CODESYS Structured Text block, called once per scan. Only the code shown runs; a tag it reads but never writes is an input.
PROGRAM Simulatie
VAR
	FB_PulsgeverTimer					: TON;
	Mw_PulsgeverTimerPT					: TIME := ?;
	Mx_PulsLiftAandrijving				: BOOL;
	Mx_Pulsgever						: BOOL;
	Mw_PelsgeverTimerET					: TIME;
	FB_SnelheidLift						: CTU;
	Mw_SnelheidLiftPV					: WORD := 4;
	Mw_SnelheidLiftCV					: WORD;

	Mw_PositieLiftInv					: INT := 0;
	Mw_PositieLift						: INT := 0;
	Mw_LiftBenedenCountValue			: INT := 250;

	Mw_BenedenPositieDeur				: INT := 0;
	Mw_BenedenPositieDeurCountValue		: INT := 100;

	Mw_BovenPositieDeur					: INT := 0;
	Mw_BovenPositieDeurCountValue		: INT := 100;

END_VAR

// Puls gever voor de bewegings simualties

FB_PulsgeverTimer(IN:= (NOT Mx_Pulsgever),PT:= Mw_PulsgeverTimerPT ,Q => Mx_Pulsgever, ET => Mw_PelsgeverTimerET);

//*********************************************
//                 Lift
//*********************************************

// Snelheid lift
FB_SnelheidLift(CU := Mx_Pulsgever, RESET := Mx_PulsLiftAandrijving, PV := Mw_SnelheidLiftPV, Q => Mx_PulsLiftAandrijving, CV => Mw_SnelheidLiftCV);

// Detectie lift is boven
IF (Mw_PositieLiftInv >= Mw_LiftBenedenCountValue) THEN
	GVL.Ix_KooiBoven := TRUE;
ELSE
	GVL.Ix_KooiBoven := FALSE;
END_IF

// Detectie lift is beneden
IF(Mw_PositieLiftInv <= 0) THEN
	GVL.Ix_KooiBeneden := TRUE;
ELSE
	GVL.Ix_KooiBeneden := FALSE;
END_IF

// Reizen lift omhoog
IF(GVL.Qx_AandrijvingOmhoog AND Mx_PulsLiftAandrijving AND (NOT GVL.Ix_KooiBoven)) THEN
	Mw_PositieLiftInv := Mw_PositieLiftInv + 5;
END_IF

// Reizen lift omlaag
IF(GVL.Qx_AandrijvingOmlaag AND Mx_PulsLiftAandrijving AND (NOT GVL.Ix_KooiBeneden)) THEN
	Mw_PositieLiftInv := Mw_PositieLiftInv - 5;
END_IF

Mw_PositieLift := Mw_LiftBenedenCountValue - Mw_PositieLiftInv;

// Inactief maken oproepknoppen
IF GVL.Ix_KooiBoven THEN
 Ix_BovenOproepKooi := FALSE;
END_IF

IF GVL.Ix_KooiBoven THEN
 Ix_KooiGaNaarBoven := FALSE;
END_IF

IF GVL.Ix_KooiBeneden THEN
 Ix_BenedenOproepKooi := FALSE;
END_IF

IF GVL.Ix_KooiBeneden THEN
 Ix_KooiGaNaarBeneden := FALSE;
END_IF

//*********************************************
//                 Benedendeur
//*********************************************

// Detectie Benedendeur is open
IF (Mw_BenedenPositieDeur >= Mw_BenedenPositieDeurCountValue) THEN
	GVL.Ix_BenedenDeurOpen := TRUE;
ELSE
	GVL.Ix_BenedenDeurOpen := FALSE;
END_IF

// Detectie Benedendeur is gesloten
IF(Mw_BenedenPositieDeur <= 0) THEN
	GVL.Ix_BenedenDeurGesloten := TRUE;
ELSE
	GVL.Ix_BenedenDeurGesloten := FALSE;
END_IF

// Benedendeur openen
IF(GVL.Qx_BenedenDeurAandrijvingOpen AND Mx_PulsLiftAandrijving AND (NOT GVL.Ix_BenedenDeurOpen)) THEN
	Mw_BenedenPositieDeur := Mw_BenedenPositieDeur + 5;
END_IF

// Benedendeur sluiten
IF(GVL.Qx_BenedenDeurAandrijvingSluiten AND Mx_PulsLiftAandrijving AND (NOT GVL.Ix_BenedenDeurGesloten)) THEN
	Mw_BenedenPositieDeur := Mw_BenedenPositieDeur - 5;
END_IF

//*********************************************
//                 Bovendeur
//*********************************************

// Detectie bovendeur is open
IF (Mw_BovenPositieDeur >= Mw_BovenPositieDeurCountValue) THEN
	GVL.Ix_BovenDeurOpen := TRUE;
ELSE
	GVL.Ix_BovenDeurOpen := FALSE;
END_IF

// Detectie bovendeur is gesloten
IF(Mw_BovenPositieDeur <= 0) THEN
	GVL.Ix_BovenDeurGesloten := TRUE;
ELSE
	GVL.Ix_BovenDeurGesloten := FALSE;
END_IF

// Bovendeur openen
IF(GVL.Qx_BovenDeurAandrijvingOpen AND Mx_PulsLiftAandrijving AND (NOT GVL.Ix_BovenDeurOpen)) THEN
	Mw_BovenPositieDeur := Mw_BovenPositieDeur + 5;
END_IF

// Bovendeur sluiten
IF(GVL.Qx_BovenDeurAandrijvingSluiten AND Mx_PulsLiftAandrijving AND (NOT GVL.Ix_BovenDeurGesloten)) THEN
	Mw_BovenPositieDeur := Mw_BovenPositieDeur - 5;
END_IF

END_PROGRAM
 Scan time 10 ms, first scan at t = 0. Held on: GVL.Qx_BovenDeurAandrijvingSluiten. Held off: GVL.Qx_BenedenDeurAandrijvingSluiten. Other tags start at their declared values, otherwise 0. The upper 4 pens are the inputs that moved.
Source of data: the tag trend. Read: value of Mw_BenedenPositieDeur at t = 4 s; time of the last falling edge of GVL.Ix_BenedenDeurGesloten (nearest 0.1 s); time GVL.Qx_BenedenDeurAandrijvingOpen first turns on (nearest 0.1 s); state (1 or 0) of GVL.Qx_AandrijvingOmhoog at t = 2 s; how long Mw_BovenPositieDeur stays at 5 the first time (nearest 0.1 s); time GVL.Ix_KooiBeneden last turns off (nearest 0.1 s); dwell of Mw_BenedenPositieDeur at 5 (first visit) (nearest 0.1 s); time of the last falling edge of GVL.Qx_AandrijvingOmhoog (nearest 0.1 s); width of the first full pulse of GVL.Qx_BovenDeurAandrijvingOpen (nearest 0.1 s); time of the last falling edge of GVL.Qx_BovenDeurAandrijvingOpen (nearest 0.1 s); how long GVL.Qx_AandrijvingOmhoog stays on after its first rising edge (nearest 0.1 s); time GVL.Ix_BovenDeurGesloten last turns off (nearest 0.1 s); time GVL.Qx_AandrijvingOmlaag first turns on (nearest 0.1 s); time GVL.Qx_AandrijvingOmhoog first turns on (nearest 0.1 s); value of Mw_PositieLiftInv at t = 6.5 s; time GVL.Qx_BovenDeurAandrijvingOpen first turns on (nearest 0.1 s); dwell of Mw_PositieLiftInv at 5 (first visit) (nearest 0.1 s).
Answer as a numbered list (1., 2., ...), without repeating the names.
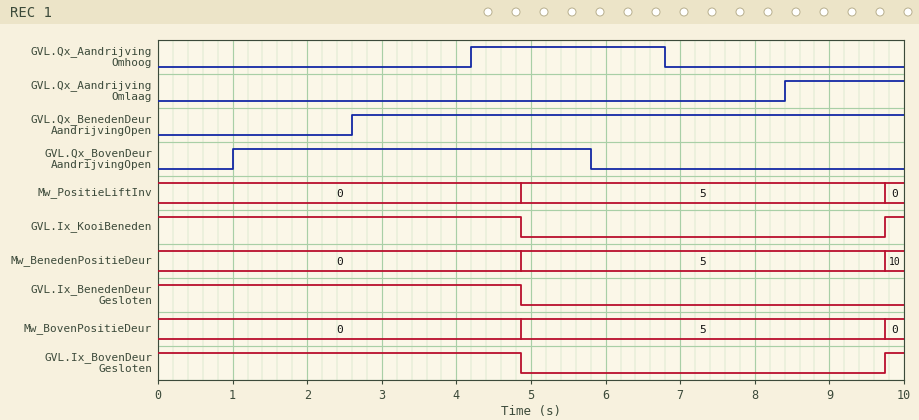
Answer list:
1. 0
2. 4.9 s
3. 2.6 s
4. 0
5. 4.9 s
6. 4.9 s
7. 4.9 s
8. 6.8 s
9. 4.8 s
10. 5.8 s
11. 2.6 s
12. 4.9 s
13. 8.4 s
14. 4.2 s
15. 5
16. 1.0 s
17. 4.9 s
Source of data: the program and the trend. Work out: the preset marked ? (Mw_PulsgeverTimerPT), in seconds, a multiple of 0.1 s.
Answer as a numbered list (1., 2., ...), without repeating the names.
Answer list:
1. 1.2 s
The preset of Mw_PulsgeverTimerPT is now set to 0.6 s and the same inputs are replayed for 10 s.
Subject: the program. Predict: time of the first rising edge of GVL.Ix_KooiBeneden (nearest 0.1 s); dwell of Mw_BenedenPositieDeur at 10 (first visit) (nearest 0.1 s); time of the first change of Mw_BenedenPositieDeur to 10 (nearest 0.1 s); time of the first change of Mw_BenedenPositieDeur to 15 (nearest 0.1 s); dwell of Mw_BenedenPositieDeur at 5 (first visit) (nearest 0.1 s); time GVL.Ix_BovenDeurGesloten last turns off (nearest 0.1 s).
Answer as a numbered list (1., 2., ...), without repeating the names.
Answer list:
1. 9.9 s
2. 2.5 s
3. 7.4 s
4. 9.9 s
5. 2.5 s
6. 2.5 s
